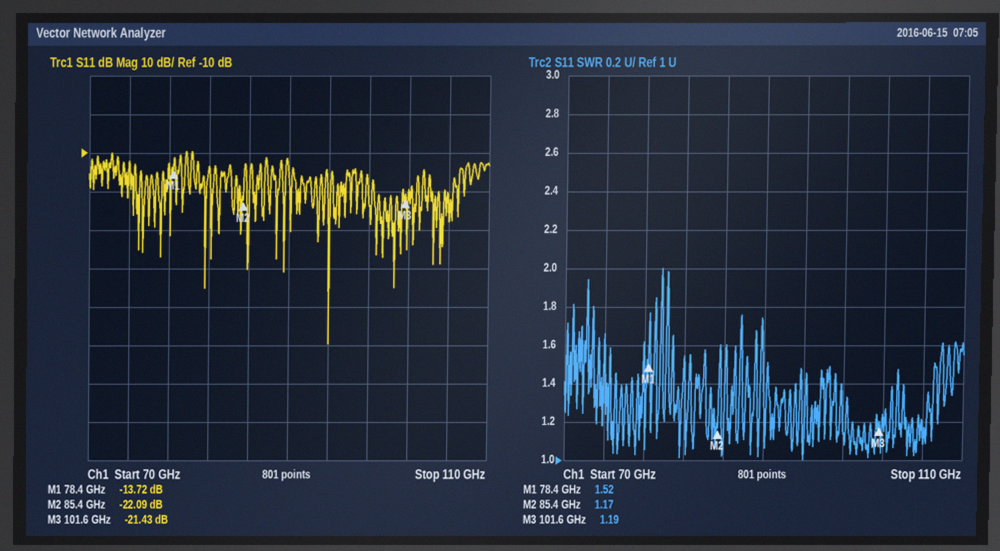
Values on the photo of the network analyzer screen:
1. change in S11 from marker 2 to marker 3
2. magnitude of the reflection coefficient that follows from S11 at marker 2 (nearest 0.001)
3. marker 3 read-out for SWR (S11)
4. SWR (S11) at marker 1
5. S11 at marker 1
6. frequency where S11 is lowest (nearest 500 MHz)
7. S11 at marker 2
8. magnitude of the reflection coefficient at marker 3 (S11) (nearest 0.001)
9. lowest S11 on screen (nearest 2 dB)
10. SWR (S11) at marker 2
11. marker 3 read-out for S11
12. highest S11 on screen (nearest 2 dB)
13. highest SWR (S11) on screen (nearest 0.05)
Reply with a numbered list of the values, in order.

1. 0.66 dB
2. 0.079
3. 1.19
4. 1.52
5. -13.72 dB
6. 94.0 GHz
7. -22.09 dB
8. 0.085
9. -60 dB
10. 1.17
11. -21.43 dB
12. -10 dB
13. 2.00
